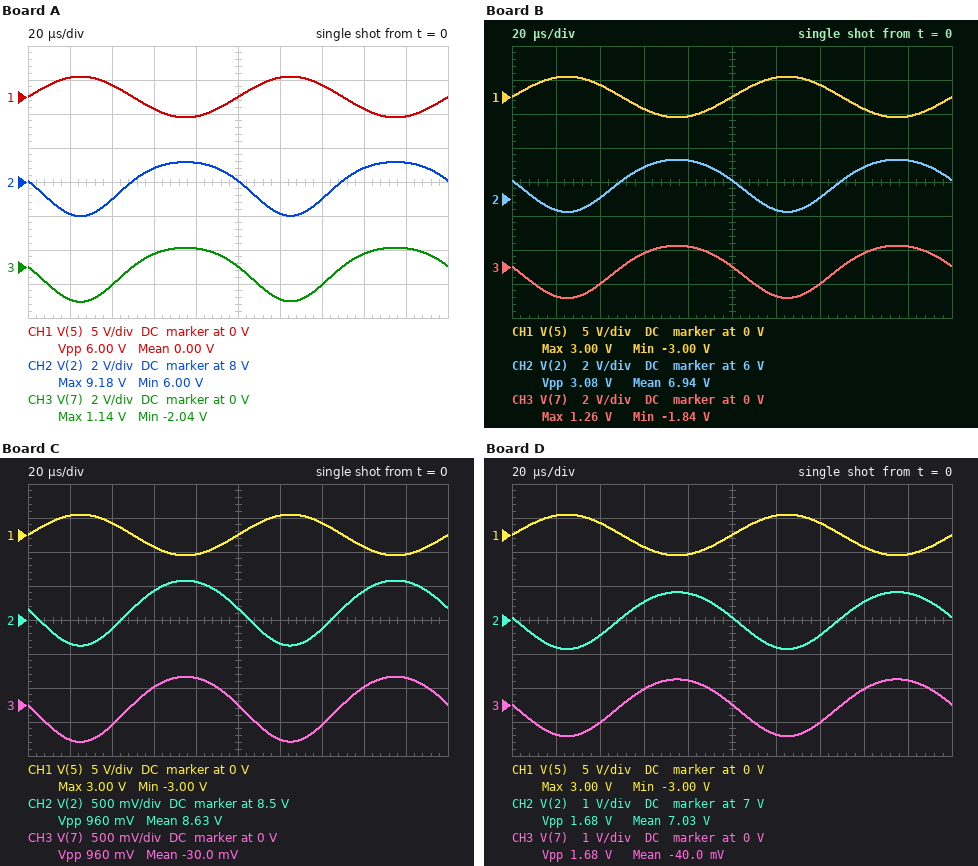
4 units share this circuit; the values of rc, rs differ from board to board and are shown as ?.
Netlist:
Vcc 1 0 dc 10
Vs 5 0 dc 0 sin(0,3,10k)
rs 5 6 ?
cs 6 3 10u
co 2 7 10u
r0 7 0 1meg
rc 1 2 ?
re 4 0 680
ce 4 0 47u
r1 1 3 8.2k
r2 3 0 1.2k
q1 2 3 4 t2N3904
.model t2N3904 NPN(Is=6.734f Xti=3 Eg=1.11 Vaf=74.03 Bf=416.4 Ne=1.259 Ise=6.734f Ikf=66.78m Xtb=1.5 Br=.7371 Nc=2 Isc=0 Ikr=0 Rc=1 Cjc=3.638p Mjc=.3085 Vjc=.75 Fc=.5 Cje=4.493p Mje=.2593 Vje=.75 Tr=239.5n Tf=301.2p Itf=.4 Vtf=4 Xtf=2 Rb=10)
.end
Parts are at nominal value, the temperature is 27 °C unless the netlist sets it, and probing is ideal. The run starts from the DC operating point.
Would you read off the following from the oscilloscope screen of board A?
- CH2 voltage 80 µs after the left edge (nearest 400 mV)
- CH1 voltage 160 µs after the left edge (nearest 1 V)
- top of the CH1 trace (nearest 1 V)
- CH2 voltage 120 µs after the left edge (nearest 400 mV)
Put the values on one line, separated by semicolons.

9.2 V; -2 V; 3 V; 6.0 V
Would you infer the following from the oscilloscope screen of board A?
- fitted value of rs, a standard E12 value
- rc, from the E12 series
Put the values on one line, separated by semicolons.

120 kΩ; 2.2 kΩ
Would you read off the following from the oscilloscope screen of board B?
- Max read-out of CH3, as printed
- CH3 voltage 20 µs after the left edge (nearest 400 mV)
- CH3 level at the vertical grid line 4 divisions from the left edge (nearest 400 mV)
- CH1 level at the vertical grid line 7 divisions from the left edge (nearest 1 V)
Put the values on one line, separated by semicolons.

1.26 V; -1.6 V; 1.2 V; 2 V
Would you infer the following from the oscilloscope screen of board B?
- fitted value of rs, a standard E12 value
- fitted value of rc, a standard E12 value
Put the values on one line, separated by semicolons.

180 kΩ; 3.3 kΩ
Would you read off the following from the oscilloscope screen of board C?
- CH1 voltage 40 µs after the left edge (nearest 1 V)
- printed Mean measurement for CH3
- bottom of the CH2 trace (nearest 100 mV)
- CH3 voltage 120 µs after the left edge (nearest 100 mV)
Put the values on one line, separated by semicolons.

2 V; -30.0 mV; 8.1 V; -500 mV
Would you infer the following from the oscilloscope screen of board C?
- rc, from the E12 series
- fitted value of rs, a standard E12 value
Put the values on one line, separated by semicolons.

1.5 kΩ; 270 kΩ
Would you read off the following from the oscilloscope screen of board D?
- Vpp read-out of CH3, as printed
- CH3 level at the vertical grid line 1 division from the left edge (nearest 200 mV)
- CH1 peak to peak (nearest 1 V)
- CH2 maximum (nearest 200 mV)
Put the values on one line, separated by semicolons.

1.68 V; -800 mV; 6 V; 7.8 V
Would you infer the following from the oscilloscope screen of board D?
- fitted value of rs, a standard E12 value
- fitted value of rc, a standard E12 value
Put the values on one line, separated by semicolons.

330 kΩ; 3.3 kΩ
